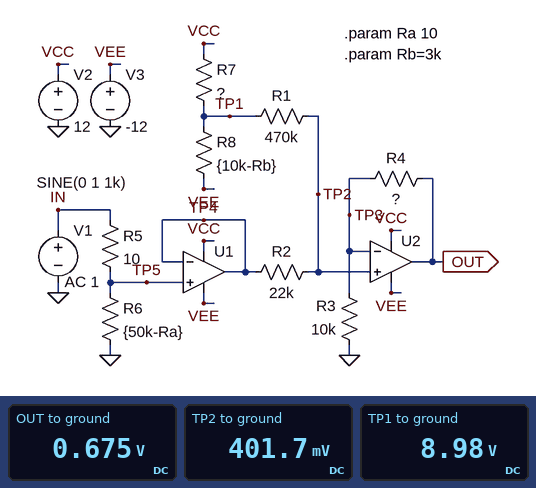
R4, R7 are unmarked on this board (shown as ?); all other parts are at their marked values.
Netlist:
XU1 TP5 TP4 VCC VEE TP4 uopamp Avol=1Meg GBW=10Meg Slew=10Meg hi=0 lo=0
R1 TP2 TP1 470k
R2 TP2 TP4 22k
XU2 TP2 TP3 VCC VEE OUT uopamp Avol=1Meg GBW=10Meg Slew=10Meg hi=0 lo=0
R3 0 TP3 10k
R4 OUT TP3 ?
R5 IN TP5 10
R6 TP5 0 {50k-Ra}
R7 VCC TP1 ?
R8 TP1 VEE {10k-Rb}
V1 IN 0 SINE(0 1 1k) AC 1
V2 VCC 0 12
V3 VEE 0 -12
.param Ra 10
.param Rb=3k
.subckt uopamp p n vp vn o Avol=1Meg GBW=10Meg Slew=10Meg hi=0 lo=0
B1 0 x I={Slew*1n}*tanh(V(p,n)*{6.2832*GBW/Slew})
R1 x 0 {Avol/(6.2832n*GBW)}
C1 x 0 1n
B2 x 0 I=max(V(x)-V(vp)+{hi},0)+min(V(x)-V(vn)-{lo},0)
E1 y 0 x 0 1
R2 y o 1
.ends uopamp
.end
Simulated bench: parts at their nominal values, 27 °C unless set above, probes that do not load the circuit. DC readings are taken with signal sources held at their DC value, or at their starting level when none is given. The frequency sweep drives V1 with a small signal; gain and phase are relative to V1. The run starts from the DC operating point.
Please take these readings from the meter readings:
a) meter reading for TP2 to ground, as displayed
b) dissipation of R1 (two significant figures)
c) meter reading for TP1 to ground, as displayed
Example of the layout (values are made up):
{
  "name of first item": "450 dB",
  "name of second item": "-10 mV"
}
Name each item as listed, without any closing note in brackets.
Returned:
{
  "meter reading for TP2 to ground, as displayed": "401.7 mV",
  "dissipation of R1": "160 µW",
  "meter reading for TP1 to ground, as displayed": "8.98 V"
}
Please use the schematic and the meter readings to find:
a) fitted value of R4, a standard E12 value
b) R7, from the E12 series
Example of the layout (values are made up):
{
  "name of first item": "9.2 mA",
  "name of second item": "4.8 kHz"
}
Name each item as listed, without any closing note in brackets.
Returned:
{
  "fitted value of R4, a standard E12 value": "6.8 kΩ",
  "R7, from the E12 series": "1 kΩ"
}
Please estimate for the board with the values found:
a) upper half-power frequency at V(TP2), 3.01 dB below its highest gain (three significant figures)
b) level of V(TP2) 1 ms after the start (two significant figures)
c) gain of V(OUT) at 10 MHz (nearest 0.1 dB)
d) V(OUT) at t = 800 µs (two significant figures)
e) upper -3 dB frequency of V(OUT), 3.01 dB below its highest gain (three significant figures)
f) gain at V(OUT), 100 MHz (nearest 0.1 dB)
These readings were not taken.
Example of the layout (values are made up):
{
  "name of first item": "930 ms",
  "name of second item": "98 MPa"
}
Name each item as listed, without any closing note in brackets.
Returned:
{
  "upper half-power frequency at V(TP2), 3.01 dB below its highest gain": "10.0 MHz",
  "level of V(TP2) 1 ms after the start": "400 mV",
  "gain of V(OUT) at 10 MHz": "-4.7 dB",
  "V(OUT) at t = 800 µs": "-850 mV",
  "upper -3 dB frequency of V(OUT), 3.01 dB below its highest gain": "4.74 MHz",
  "gain at V(OUT), 100 MHz": "-40.5 dB"
}
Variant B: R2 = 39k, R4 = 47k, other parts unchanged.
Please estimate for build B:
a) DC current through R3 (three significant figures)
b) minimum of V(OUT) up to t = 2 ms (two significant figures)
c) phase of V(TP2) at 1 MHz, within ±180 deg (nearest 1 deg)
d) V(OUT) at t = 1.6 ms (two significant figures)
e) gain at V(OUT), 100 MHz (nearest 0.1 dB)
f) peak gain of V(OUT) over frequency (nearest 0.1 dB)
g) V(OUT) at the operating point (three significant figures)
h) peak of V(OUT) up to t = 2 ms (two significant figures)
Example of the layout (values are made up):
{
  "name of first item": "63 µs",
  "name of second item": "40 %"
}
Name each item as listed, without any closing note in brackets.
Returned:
{
  "DC current through R3": "68.8 µA",
  "minimum of V(OUT) up to t = 2 ms": "-1.3 V",
  "phase of V(TP2) at 1 MHz, within ±180 deg": "-6 deg",
  "V(OUT) at t = 1.6 ms": "830 mV",
  "gain at V(OUT), 100 MHz": "-40.7 dB",
  "peak gain of V(OUT) over frequency": "14.4 dB",
  "V(OUT) at the operating point": "3.92 V",
  "peak of V(OUT) up to t = 2 ms": "9.2 V"
}
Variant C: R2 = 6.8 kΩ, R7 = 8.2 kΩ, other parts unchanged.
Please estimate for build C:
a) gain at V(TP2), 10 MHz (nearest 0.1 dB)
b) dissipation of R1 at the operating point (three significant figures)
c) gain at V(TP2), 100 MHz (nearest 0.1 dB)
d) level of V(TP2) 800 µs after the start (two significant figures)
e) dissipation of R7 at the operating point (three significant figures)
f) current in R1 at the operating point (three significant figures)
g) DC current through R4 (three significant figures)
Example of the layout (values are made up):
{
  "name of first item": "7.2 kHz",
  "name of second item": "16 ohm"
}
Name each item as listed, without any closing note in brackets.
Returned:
{
  "gain at V(TP2), 10 MHz": "-3.1 dB",
  "dissipation of R1 at the operating point": "1.83 µW",
  "gain at V(TP2), 100 MHz": "-20.2 dB",
  "level of V(TP2) 800 µs after the start": "-950 mV",
  "dissipation of R7 at the operating point": "20.4 mW",
  "current in R1 at the operating point": "1.97 µA",
  "DC current through R4": "1.34 µA"
}
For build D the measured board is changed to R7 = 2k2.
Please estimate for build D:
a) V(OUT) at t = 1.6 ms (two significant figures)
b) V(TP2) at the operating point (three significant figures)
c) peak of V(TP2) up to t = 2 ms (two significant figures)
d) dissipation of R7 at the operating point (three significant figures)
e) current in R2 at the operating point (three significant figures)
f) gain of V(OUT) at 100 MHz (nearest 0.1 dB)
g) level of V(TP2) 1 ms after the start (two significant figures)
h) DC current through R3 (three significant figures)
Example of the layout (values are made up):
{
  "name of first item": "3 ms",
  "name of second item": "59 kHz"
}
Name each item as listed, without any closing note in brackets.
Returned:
{
  "V(OUT) at t = 1.6 ms": "-470 mV",
  "V(TP2) at the operating point": "279 mV",
  "peak of V(TP2) up to t = 2 ms": "1.2 V",
  "dissipation of R7 at the operating point": "15.1 mW",
  "current in R2 at the operating point": "12.7 µA",
  "gain of V(OUT) at 100 MHz": "-40.5 dB",
  "level of V(TP2) 1 ms after the start": "280 mV",
  "DC current through R3": "27.9 µA"
}
